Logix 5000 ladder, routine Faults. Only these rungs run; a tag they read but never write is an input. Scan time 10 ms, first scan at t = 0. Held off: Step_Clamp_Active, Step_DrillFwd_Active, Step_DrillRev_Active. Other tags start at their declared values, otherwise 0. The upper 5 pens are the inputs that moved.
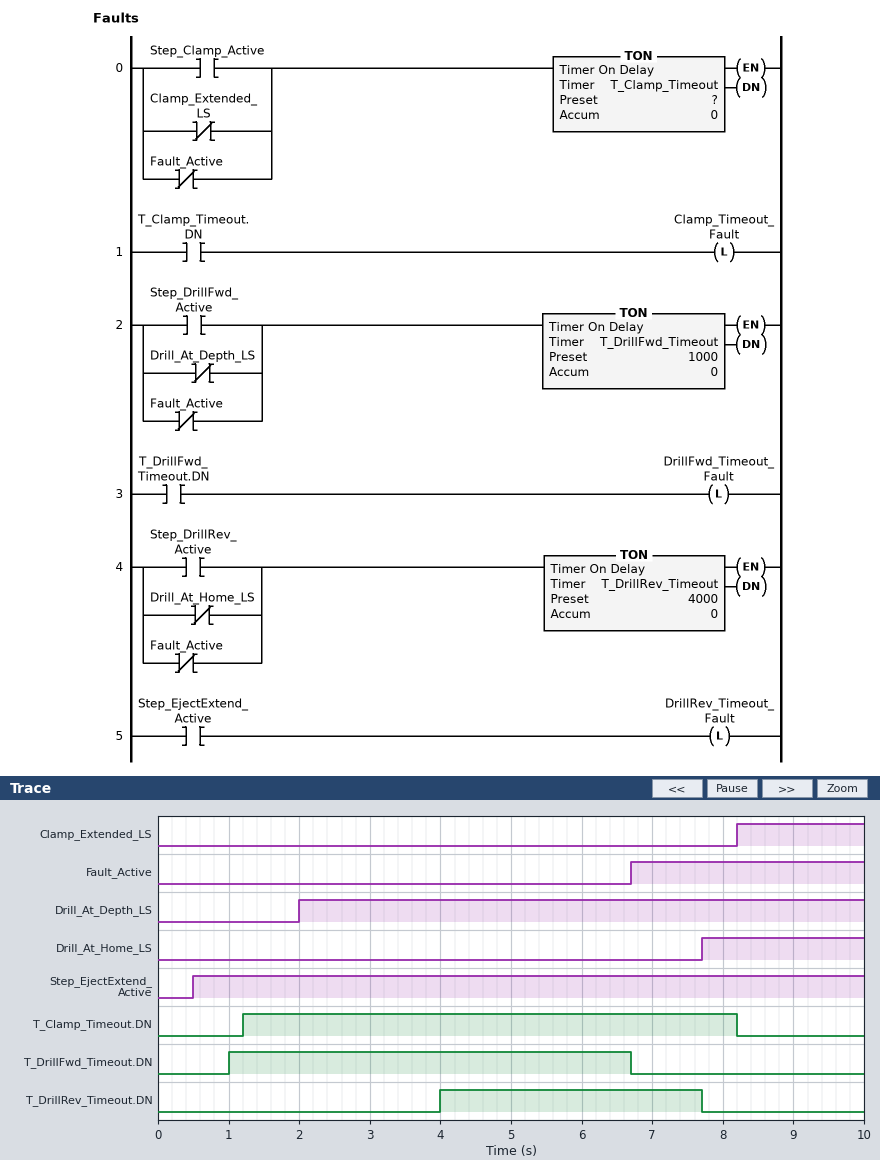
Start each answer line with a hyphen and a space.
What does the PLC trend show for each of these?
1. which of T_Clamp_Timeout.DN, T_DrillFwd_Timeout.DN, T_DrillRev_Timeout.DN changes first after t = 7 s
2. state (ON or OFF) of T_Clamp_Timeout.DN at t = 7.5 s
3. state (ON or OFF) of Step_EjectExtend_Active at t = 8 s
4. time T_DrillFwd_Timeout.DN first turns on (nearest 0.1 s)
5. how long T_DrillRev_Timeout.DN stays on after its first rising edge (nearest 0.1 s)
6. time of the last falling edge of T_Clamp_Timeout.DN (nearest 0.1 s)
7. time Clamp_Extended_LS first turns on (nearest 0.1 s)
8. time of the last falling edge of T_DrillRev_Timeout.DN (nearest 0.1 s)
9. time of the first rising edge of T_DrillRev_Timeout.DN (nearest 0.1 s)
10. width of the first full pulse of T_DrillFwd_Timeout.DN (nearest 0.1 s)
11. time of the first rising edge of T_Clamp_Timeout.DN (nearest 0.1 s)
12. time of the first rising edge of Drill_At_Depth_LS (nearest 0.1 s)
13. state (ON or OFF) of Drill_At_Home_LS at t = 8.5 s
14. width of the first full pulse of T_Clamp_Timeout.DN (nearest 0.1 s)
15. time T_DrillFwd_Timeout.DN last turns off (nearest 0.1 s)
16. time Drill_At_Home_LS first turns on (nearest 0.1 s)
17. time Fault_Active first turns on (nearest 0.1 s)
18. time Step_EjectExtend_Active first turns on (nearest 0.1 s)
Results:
- T_DrillRev_Timeout.DN
- ON
- ON
- 1.0 s
- 3.7 s
- 8.2 s
- 8.2 s
- 7.7 s
- 4.0 s
- 5.7 s
- 1.2 s
- 2.0 s
- ON
- 7.0 s
- 6.7 s
- 7.7 s
- 6.7 s
- 0.5 s
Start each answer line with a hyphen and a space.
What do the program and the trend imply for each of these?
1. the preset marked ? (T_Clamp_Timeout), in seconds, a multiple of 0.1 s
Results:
- 1.2 s
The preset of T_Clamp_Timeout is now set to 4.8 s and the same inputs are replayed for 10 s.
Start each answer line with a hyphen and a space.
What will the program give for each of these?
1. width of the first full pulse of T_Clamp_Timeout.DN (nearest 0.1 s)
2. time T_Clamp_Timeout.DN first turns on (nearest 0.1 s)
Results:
- 3.4 s
- 4.8 s
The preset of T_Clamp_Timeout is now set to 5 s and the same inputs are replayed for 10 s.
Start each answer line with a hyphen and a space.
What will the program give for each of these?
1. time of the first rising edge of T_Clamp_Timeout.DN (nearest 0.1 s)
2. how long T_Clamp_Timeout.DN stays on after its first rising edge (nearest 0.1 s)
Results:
- 5.0 s
- 3.2 s
